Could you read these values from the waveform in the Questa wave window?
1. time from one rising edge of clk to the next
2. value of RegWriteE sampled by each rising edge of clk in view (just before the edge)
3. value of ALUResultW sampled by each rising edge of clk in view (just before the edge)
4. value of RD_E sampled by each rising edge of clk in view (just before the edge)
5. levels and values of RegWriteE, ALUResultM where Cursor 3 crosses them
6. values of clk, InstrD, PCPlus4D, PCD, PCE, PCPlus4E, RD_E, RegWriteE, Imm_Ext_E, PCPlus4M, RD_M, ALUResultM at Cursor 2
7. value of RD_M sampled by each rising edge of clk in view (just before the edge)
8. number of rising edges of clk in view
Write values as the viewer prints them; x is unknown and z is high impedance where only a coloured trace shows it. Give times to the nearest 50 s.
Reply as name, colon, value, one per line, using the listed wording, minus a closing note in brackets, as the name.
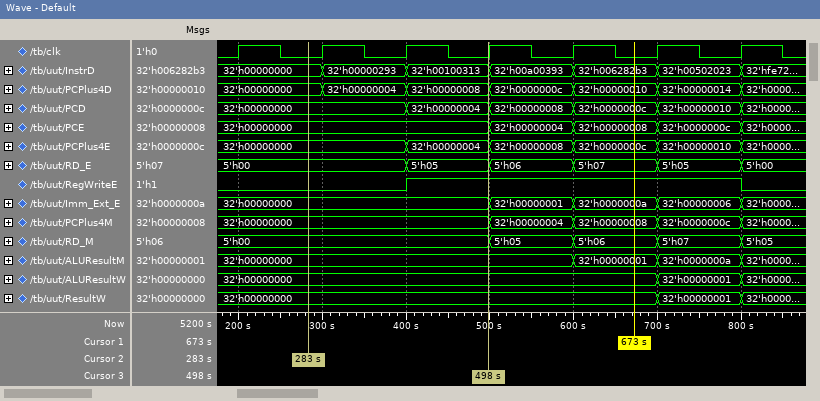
time from one rising edge of clk to the next: 100 s
value of RegWriteE sampled by each rising edge of clk in view: 0 0 0 1 1 1 1
value of ALUResultW sampled by each rising edge of clk in view: 32'h00000000, 32'h00000000, 32'h00000000, 32'h00000000, 32'h00000000, 32'h00000000, 32'h00000001
value of RD_E sampled by each rising edge of clk in view: 5'h00, 5'h00, 5'h00, 5'h05, 5'h06, 5'h07, 5'h05
levels and values of RegWriteE, ALUResultM where Cursor 3 crosses them: RegWriteE=1, ALUResultM=32'h00000000
values of clk, InstrD, PCPlus4D, PCD, PCE, PCPlus4E, RD_E, RegWriteE, Imm_Ext_E, PCPlus4M, RD_M, ALUResultM at Cursor 2: clk=0, InstrD=32'h00000000, PCPlus4D=32'h00000000, PCD=32'h00000000, PCE=32'h00000000, PCPlus4E=32'h00000000, RD_E=5'h00, RegWriteE=0, Imm_Ext_E=32'h00000000, PCPlus4M=32'h00000000, RD_M=5'h00, ALUResultM=32'h00000000
value of RD_M sampled by each rising edge of clk in view: 5'h00, 5'h00, 5'h00, 5'h00, 5'h05, 5'h06, 5'h07
number of rising edges of clk in view: 7
